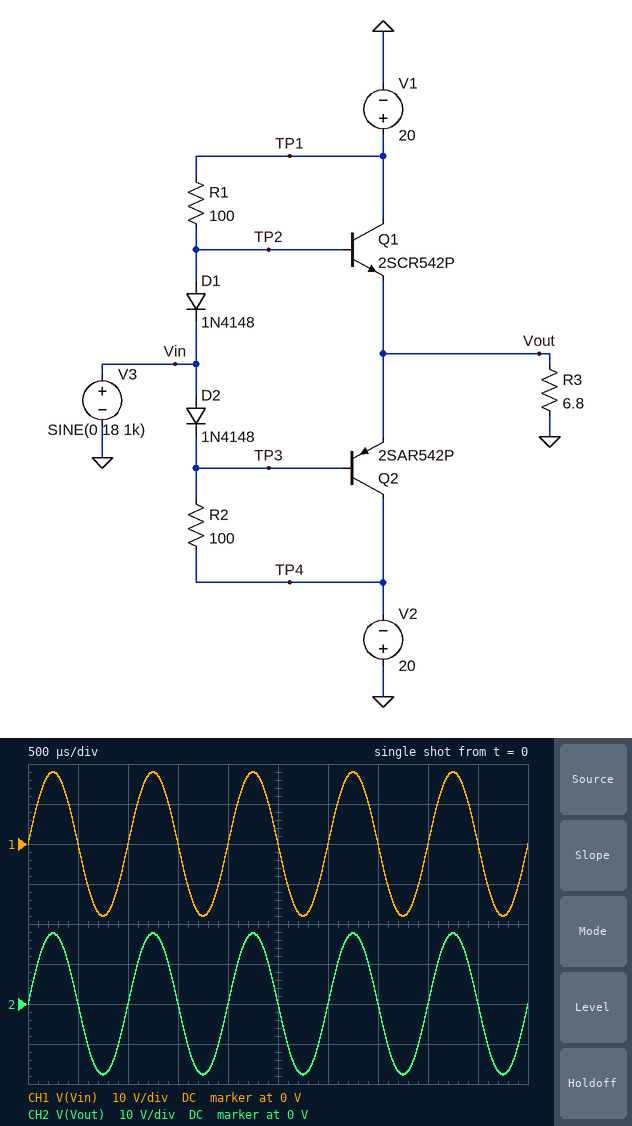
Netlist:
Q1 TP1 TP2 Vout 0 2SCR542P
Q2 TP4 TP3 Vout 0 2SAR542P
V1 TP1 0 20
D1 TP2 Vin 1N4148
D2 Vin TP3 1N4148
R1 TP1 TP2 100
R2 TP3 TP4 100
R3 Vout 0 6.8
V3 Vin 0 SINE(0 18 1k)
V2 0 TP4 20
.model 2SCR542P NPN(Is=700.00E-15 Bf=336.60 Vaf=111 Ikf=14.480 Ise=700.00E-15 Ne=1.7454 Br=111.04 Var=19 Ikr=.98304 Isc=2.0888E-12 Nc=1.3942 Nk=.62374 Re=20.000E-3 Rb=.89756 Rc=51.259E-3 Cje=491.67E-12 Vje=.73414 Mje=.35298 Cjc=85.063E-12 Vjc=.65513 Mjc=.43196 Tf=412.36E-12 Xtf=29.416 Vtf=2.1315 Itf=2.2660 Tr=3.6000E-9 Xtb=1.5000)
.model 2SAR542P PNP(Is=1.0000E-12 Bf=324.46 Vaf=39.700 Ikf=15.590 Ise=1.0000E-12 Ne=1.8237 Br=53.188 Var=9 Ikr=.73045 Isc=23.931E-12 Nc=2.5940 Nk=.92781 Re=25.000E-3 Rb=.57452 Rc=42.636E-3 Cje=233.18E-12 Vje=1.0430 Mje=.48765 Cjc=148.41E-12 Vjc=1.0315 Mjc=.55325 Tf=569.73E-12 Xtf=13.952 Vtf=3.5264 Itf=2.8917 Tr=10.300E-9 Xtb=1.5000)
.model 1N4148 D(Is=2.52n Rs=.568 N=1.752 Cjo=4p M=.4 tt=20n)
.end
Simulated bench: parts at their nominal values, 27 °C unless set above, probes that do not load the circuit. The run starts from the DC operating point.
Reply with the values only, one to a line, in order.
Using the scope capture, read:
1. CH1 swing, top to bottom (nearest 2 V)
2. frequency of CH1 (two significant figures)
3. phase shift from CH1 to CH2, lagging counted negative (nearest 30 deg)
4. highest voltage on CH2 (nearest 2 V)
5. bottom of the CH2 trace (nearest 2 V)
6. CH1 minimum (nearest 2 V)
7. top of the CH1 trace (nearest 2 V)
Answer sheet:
36 V
1.0 kHz
0 deg
18 V
-18 V
-18 V
18 V
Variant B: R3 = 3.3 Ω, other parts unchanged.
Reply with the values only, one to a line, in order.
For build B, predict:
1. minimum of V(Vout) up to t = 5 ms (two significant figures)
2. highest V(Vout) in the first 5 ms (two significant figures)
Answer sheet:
-16 V
17 V
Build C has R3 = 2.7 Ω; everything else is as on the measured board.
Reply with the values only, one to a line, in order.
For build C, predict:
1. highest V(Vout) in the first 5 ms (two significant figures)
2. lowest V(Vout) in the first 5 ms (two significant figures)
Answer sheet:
16 V
-15 V
